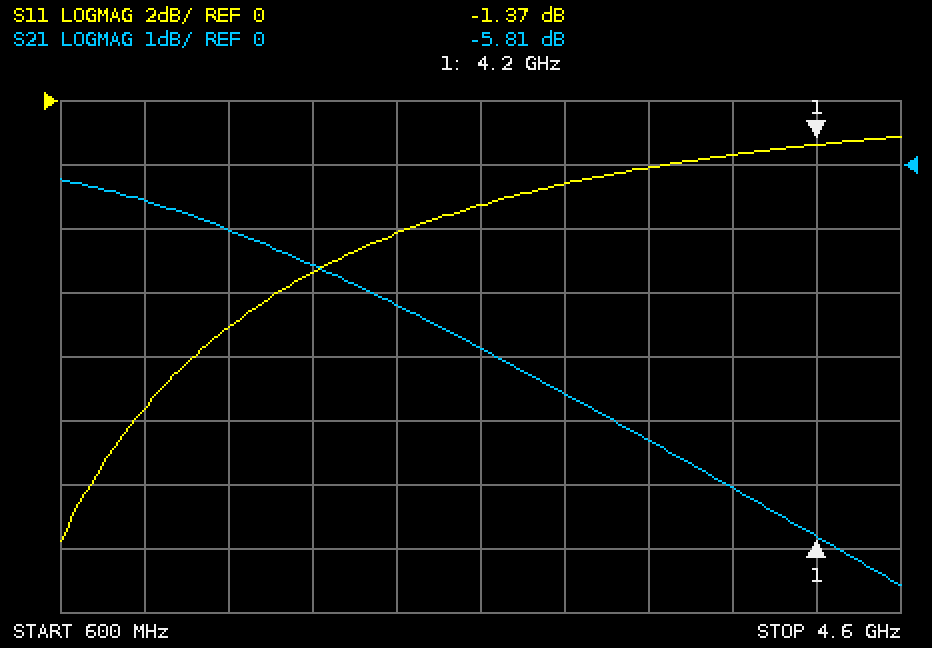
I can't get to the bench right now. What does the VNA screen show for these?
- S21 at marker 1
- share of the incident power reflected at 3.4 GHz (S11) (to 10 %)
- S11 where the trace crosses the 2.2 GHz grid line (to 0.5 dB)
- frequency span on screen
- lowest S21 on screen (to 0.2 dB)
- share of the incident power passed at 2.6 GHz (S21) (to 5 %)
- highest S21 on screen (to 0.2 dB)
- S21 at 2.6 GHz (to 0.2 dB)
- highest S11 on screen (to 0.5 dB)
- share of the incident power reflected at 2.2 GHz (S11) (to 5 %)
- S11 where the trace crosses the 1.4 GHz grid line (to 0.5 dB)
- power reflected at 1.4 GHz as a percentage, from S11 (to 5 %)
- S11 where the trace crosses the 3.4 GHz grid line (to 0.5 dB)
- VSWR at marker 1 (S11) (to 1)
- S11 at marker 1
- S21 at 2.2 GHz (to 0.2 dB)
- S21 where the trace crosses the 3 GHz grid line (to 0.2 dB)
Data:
-5.81 dB
60 %
-4.0 dB
4 GHz
-6.6 dB
50 %
-0.2 dB
-2.8 dB
-1.0 dB
40 %
-7.0 dB
20 %
-2.0 dB
13
-1.37 dB
-2.2 dB
-3.6 dB
